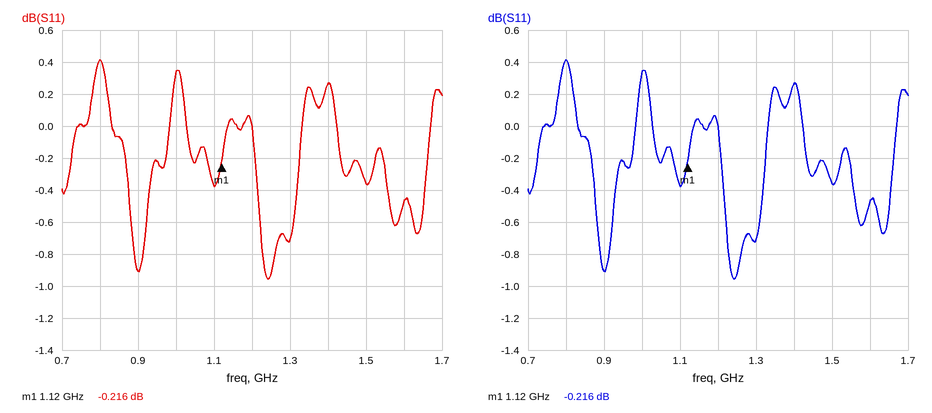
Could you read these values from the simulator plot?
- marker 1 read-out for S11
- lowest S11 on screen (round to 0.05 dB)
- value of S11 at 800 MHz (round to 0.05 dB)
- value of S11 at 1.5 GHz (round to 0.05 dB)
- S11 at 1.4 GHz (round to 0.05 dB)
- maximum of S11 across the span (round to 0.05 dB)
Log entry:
-0.216 dB
-0.95 dB
0.40 dB
-0.35 dB
0.25 dB
0.40 dB
